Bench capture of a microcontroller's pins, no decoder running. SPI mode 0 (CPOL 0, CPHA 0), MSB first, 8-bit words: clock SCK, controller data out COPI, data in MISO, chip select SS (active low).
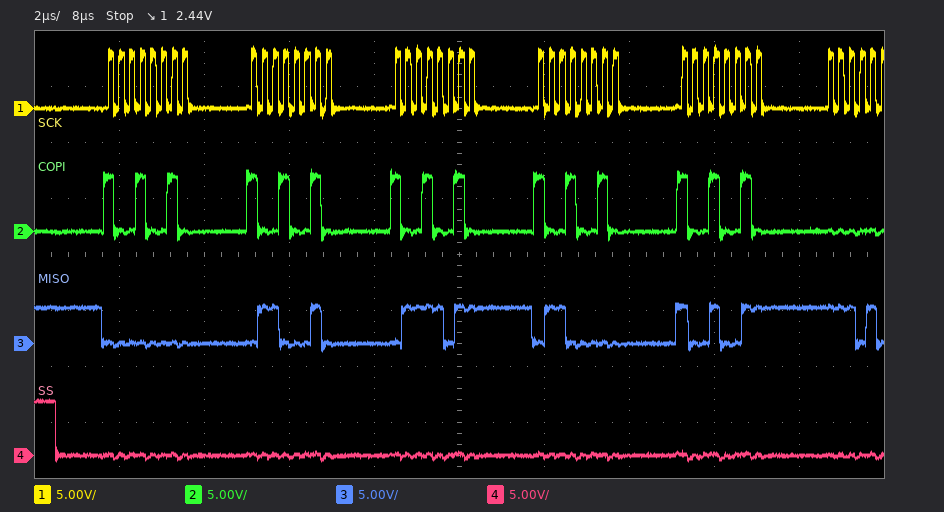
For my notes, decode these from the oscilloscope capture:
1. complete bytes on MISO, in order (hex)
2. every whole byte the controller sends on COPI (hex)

00 62 7B 60 93
92 92 92 92 92
